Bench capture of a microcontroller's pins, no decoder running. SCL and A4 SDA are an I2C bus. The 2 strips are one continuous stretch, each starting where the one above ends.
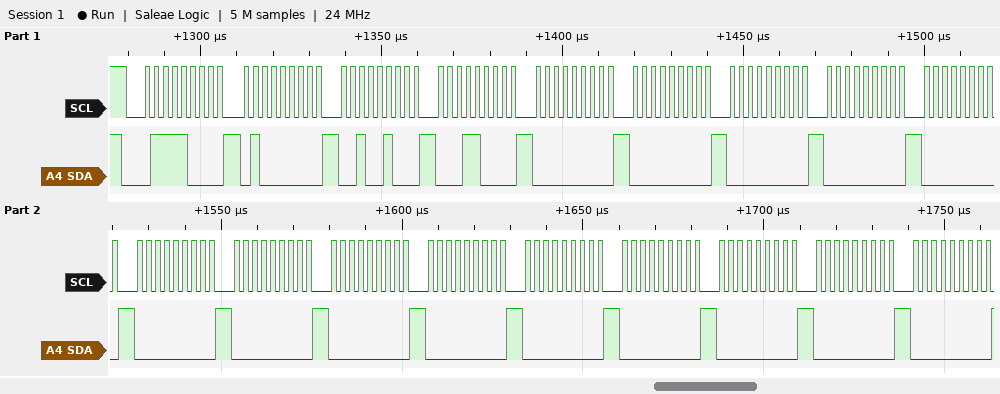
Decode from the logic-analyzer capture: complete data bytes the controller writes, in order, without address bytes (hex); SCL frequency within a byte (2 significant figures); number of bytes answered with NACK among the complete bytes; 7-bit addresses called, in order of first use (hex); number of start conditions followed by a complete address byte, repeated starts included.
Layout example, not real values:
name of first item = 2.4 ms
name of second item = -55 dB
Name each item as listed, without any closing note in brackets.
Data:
complete data bytes the controller writes, in order, without address bytes = 40 24 18 00 00 00 00 00 00 00 00 00 00 00 00 00 00
SCL frequency within a byte = 400 kHz
number of bytes answered with NACK among the complete bytes = 0
7-bit addresses called, in order of first use = 0x3C
number of start conditions followed by a complete address byte, repeated starts included = 1
